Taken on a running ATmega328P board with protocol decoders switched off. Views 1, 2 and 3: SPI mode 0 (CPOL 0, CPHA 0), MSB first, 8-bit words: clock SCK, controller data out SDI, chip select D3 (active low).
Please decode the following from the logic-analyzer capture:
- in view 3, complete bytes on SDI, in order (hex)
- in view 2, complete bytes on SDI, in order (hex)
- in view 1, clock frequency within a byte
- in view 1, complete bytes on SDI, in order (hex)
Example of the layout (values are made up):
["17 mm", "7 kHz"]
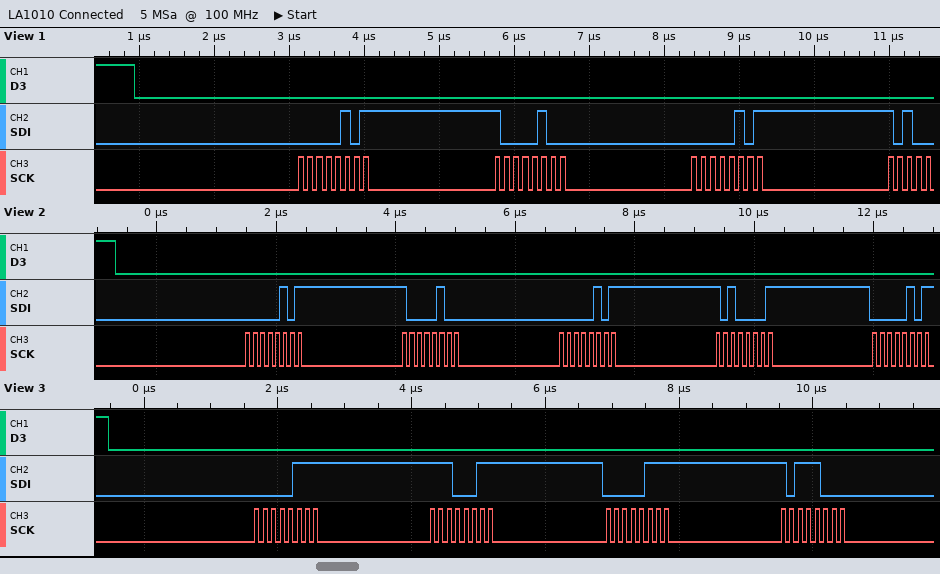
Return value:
["07 E3 07 B8", "05 84 05 A1 05", "8 MHz", "0x05 0x84 0x05"]
